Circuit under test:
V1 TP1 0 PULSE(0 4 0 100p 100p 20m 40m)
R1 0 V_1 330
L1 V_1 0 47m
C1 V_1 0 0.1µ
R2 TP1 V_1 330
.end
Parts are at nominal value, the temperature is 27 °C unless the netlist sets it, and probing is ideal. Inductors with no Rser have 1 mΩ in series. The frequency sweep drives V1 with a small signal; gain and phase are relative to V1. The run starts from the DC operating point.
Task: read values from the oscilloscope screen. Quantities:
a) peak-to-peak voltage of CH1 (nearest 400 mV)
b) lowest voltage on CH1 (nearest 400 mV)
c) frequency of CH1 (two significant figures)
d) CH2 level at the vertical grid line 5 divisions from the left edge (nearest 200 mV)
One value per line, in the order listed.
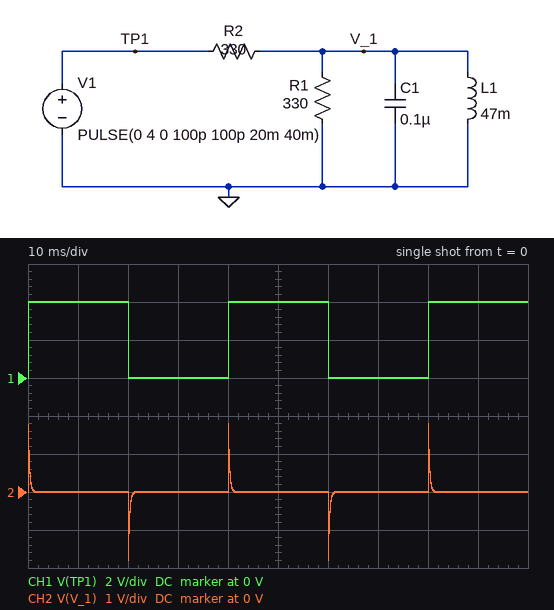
4.0 V
0 V
25 Hz
0 V
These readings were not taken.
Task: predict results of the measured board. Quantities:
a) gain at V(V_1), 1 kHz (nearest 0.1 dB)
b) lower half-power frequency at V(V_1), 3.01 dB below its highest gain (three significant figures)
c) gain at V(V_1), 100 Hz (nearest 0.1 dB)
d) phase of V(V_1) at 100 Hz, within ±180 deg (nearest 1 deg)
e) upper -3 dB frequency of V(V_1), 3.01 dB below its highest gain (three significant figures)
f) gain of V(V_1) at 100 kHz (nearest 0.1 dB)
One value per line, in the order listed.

-6.8 dB
530 Hz
-21.1 dB
80 deg
10.2 kHz
-26.4 dB
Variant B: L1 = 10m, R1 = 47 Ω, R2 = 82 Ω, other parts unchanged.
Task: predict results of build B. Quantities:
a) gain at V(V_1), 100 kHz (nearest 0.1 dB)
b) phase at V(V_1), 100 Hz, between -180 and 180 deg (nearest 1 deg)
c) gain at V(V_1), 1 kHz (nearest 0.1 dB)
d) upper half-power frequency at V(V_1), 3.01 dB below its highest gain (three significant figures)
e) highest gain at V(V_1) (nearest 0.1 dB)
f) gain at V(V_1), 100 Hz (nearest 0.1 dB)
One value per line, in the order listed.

-15.3 dB
78 deg
-9.6 dB
53.7 kHz
-8.8 dB
-22.5 dB
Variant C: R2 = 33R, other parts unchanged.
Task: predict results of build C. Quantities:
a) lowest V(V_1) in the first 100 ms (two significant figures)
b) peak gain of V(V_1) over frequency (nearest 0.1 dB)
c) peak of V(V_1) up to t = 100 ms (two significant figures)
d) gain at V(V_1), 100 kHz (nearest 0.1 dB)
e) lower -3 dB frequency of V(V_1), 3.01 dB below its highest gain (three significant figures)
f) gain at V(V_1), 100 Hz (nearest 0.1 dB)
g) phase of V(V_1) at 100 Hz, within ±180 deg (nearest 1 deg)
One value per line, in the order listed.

-3.6 V
-0.8 dB
3.6 V
-7.4 dB
101 Hz
-3.9 dB
45 deg
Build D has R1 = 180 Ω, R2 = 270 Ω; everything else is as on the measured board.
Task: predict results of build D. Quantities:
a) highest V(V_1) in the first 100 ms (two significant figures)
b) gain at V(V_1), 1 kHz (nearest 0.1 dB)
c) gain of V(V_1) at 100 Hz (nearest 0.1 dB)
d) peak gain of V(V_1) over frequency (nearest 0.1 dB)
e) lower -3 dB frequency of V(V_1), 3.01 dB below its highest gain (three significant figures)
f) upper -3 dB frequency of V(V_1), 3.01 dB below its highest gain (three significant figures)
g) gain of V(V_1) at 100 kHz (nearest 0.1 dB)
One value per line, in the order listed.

1.5 V
-8.3 dB
-19.5 dB
-8.0 dB
357 Hz
15.1 kHz
-24.7 dB
